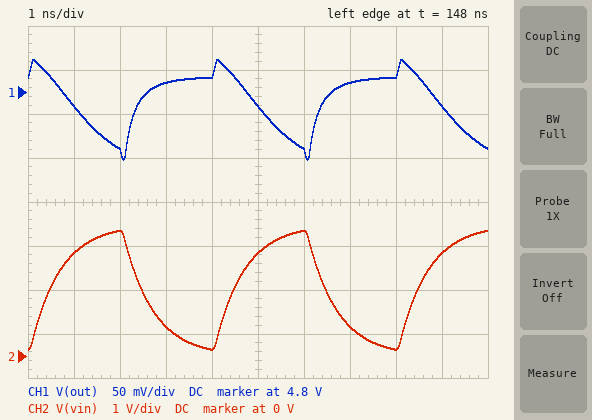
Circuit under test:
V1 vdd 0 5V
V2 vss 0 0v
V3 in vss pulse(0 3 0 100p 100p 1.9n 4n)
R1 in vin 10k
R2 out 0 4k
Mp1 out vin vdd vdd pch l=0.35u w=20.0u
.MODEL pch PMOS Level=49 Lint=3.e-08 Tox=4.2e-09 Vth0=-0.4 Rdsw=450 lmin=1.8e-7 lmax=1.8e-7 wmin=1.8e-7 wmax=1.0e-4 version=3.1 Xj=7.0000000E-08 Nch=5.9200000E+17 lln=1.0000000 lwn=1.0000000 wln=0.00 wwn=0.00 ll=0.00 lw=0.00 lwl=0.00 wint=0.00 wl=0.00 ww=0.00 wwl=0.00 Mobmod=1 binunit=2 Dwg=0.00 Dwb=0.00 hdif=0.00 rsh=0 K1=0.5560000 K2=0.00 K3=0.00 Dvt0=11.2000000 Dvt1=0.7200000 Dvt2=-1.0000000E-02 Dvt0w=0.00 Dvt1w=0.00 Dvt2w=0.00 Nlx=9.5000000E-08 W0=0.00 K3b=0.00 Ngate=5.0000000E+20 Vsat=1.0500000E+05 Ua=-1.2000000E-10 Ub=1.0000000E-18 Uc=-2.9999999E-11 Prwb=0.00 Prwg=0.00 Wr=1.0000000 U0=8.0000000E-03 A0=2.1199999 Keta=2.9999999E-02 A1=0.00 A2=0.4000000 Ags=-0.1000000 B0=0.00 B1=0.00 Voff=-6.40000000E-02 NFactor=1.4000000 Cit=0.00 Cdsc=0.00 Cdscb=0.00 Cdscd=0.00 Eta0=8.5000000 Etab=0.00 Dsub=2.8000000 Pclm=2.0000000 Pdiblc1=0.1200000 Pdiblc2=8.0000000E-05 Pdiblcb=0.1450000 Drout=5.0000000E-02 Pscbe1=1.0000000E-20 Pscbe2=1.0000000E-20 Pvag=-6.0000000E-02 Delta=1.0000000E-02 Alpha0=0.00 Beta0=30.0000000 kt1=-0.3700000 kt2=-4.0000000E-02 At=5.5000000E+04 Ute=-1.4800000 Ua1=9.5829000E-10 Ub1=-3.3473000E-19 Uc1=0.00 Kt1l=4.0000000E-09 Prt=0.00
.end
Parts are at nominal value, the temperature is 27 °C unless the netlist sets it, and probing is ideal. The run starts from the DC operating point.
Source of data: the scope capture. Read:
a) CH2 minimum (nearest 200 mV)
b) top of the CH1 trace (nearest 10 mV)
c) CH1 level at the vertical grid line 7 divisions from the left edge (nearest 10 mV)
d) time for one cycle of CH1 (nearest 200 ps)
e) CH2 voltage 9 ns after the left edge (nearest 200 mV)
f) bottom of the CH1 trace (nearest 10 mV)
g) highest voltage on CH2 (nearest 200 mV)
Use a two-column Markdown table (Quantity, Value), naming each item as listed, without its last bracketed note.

| Quantity | Value |
|---|---|
| CH2 minimum | 200 mV |
| top of the CH1 trace | 4.84 V |
| CH1 level at the vertical grid line 7 divisions from the left edge | 4.81 V |
| time for one cycle of CH1 | 4.0 ns |
| CH2 voltage 9 ns after the left edge | 2.4 V |
| bottom of the CH1 trace | 4.72 V |
| highest voltage on CH2 | 2.8 V |
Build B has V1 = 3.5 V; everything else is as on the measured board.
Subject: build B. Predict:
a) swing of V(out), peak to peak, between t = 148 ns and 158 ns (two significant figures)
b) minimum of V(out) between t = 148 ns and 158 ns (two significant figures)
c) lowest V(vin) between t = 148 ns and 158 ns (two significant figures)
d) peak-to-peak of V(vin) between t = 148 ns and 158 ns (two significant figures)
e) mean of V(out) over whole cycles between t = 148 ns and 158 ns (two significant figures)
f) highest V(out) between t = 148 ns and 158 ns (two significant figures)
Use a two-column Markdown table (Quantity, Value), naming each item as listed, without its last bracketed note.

| Quantity | Value |
|---|---|
| swing of V(out), peak to peak, between t = 148 ns and 158 ns | 2.3 V |
| minimum of V(out) between t = 148 ns and 158 ns | 1.1 V |
| lowest V(vin) between t = 148 ns and 158 ns | 160 mV |
| peak-to-peak of V(vin) between t = 148 ns and 158 ns | 2.6 V |
| mean of V(out) over whole cycles between t = 148 ns and 158 ns | 2.9 V |
| highest V(out) between t = 148 ns and 158 ns | 3.4 V |
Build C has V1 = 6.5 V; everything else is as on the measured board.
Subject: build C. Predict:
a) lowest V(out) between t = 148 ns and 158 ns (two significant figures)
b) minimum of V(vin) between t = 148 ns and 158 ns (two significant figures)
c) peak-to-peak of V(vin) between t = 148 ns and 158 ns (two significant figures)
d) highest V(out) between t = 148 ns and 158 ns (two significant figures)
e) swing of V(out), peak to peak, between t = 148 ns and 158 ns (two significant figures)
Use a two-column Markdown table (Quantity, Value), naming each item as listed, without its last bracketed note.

| Quantity | Value |
|---|---|
| lowest V(out) between t = 148 ns and 158 ns | 6.2 V |
| minimum of V(vin) between t = 148 ns and 158 ns | 130 mV |
| peak-to-peak of V(vin) between t = 148 ns and 158 ns | 2.7 V |
| highest V(out) between t = 148 ns and 158 ns | 6.3 V |
| swing of V(out), peak to peak, between t = 148 ns and 158 ns | 47 mV |
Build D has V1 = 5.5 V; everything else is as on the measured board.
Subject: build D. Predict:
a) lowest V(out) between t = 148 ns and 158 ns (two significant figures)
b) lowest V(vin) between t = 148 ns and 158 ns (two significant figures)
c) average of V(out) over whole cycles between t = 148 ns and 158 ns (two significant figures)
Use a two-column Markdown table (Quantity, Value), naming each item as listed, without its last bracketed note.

| Quantity | Value |
|---|---|
| lowest V(out) between t = 148 ns and 158 ns | 5.2 V |
| lowest V(vin) between t = 148 ns and 158 ns | 140 mV |
| average of V(out) over whole cycles between t = 148 ns and 158 ns | 5.3 V |
